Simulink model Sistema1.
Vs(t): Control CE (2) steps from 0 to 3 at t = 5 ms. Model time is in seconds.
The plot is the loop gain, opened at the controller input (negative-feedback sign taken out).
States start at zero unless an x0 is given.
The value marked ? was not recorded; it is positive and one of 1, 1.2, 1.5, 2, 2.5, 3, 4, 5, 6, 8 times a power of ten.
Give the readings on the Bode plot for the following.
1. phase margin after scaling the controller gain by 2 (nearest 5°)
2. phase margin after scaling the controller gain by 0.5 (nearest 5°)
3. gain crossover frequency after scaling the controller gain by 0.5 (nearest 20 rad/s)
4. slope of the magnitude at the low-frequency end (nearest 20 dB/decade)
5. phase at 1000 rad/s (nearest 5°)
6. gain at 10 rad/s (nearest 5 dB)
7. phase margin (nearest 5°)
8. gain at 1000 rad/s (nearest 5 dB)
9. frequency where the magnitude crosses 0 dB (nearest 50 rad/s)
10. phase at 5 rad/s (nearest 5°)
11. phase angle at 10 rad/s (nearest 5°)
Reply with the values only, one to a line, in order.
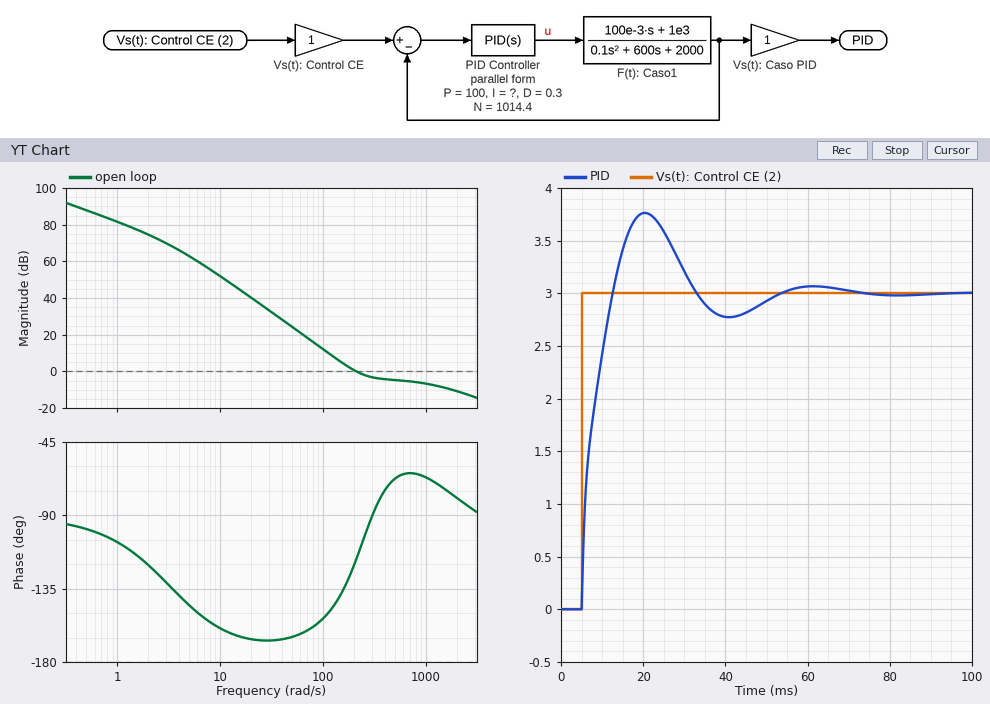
115°
40°
140 rad/s
-20 dB/decade
-65°
50 dB
65°
-5 dB
200 rad/s
-145°
-160°
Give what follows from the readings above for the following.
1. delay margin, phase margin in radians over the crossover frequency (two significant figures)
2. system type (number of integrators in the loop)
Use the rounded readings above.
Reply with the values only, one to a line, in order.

0.0057 s
1
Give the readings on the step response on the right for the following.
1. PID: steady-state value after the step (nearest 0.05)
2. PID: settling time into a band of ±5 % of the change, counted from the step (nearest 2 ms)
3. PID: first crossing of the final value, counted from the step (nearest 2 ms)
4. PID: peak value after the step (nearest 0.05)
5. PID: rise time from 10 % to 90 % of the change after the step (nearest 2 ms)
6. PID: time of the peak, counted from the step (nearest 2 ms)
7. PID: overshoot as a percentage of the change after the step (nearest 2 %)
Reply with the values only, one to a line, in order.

3.00
42 ms
8 ms
3.75
6 ms
16 ms
26 %
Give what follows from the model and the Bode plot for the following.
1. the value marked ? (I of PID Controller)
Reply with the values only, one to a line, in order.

25000
